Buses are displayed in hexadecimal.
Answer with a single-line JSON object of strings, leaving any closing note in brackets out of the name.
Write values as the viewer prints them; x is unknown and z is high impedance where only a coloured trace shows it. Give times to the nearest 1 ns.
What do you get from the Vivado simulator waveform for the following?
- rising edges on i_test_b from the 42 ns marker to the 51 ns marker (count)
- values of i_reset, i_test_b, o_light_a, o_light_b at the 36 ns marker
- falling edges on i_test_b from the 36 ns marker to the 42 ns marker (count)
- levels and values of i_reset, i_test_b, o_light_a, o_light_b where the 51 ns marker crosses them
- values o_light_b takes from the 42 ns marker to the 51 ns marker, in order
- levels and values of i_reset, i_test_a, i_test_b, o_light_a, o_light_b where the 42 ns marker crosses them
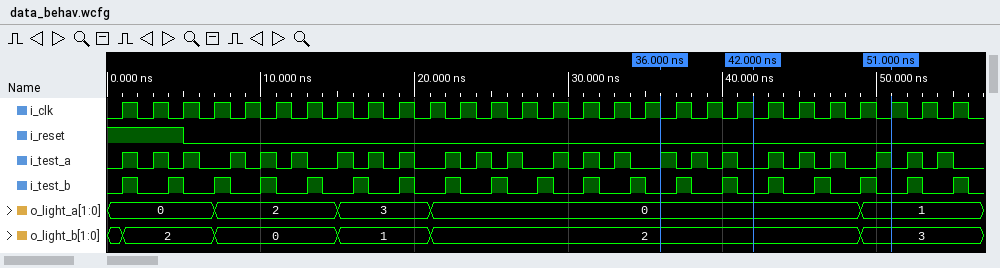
{"rising edges on i_test_b from the 42 ns marker to the 51 ns marker": "3", "values of i_reset, i_test_b, o_light_a, o_light_b at the 36 ns marker": "i_reset=0, i_test_b=0, o_light_a=0, o_light_b=2", "falling edges on i_test_b from the 36 ns marker to the 42 ns marker": "2", "levels and values of i_reset, i_test_b, o_light_a, o_light_b where the 51 ns marker crosses them": "i_reset=0, i_test_b=0, o_light_a=1, o_light_b=3", "values o_light_b takes from the 42 ns marker to the 51 ns marker, in order": "2, 3", "levels and values of i_reset, i_test_a, i_test_b, o_light_a, o_light_b where the 42 ns marker crosses them": "i_reset=0, i_test_a=0, i_test_b=0, o_light_a=0, o_light_b=2"}
